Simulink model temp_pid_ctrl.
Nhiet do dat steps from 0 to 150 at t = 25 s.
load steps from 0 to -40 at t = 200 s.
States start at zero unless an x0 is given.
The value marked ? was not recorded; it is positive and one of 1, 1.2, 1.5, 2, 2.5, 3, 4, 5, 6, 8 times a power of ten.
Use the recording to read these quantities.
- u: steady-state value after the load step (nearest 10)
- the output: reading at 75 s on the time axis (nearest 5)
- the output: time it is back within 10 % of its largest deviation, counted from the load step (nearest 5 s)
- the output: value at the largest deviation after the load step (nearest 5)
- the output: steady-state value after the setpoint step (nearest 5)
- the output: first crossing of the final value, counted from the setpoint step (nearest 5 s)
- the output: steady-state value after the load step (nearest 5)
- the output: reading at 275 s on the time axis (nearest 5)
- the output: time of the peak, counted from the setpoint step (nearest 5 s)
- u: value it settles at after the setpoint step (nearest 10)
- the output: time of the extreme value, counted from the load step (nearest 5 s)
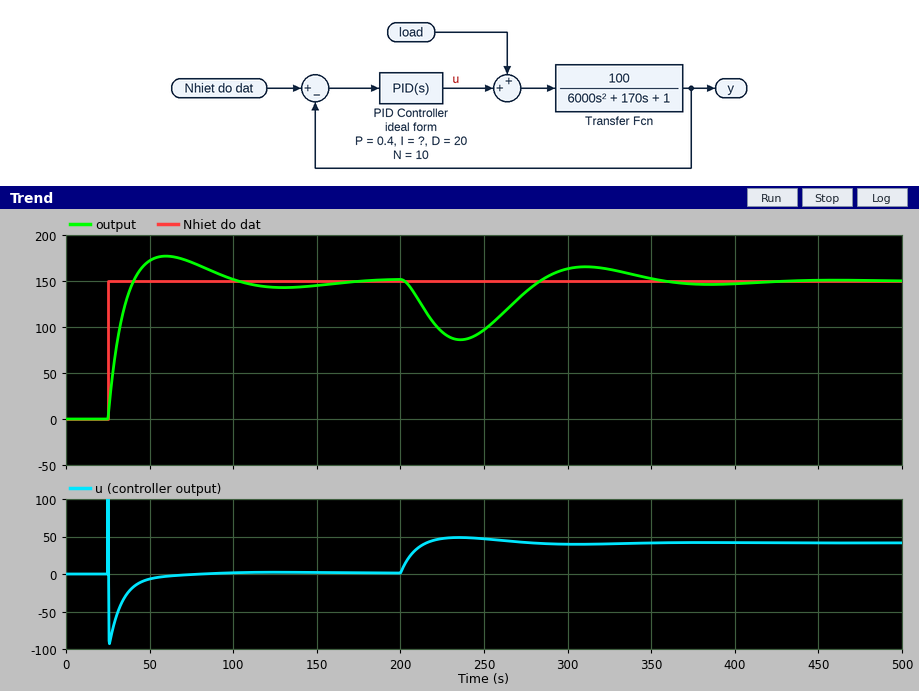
40
170
140 s
85
150
15 s
150
140
35 s
0
35 s
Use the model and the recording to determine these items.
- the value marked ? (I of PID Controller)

0.04
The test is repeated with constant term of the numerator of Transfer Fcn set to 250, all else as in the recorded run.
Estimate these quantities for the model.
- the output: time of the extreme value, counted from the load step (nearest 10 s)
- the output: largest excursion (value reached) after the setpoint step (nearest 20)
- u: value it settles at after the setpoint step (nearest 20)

30 s
160
0
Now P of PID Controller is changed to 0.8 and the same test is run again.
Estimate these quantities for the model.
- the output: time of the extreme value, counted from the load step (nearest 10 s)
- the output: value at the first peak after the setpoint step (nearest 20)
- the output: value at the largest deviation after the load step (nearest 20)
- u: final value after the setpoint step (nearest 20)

30 s
160
120
0
